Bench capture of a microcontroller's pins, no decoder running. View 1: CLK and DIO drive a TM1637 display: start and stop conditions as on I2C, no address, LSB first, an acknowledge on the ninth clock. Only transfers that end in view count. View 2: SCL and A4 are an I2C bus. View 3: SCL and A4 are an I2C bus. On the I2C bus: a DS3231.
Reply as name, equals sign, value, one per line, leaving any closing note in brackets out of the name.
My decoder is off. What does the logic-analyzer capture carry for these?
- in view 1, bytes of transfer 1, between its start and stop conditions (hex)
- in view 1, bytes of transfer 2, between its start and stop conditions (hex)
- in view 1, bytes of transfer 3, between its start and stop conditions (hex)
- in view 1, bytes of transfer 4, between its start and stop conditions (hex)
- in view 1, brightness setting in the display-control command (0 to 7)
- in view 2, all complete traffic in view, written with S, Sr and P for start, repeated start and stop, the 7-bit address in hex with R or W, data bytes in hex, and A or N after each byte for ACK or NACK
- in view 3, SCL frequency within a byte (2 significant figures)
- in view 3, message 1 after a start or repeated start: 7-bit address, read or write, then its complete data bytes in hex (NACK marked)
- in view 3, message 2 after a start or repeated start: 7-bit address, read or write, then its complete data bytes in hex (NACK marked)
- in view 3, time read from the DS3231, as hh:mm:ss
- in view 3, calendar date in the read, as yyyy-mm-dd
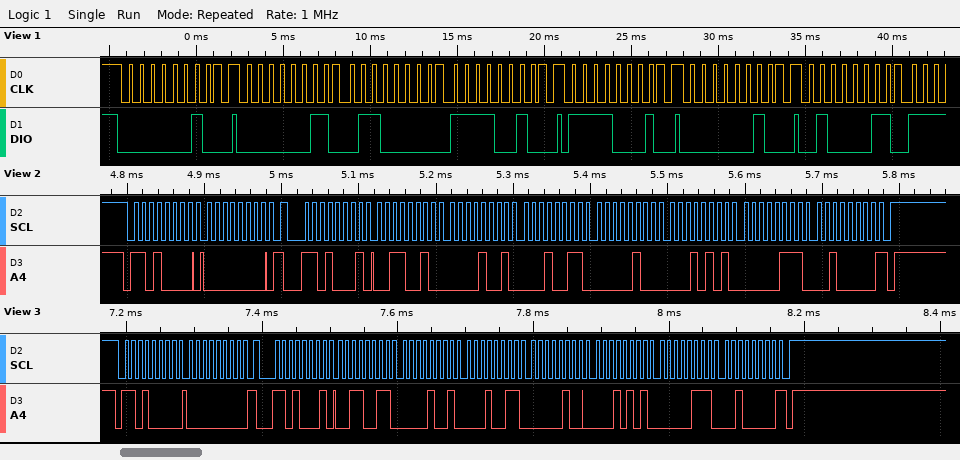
in view 1, bytes of transfer 1, between its start and stop conditions = 40
in view 1, bytes of transfer 2, between its start and stop conditions = C0 06 4F
in view 1, bytes of transfer 3, between its start and stop conditions = 8F
in view 1, bytes of transfer 4, between its start and stop conditions = 40
in view 1, brightness setting in the display-control command = 7
in view 2, all complete traffic in view, written with S, Sr and P for start, repeated start and stop, the 7-bit address in hex with R or W, data bytes in hex, and A or N after each byte for ACK or NACK = S 68W A 00 A Sr 68R A 32 A 09 A 13 A 04 A 15 A 07 A 20 N P
in view 3, SCL frequency within a byte = 100 kHz
in view 3, message 1 after a start or repeated start: 7-bit address, read or write, then its complete data bytes in hex = 0x68 write: 00
in view 3, message 2 after a start or repeated start: 7-bit address, read or write, then its complete data bytes in hex = 0x68 read: 33 09 13 04 15 07 20 NACK
in view 3, time read from the DS3231, as hh:mm:ss = 13:09:33
in view 3, calendar date in the read, as yyyy-mm-dd = 2020-07-15
